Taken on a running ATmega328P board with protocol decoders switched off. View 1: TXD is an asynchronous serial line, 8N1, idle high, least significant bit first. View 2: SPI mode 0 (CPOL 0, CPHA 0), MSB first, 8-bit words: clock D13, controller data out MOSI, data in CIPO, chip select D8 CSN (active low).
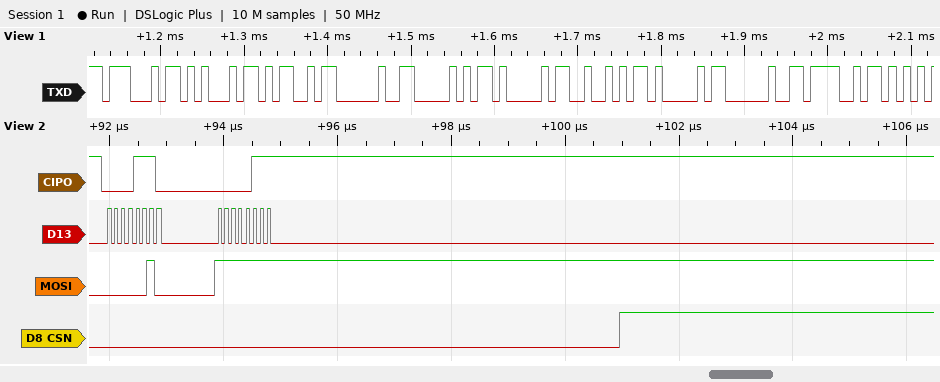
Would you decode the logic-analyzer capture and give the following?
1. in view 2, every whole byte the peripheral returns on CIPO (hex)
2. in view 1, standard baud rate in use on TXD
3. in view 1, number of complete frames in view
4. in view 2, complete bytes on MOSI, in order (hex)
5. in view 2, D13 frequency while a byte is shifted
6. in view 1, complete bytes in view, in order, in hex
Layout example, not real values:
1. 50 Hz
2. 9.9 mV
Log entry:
1. 0E 07
2. 115200 baud
3. 10
4. 02 FF
5. 8 MHz
6. 0x47 0x45 0x4D 0x20 0x50 0x41 0x52 0x41 0x20 0x4F
